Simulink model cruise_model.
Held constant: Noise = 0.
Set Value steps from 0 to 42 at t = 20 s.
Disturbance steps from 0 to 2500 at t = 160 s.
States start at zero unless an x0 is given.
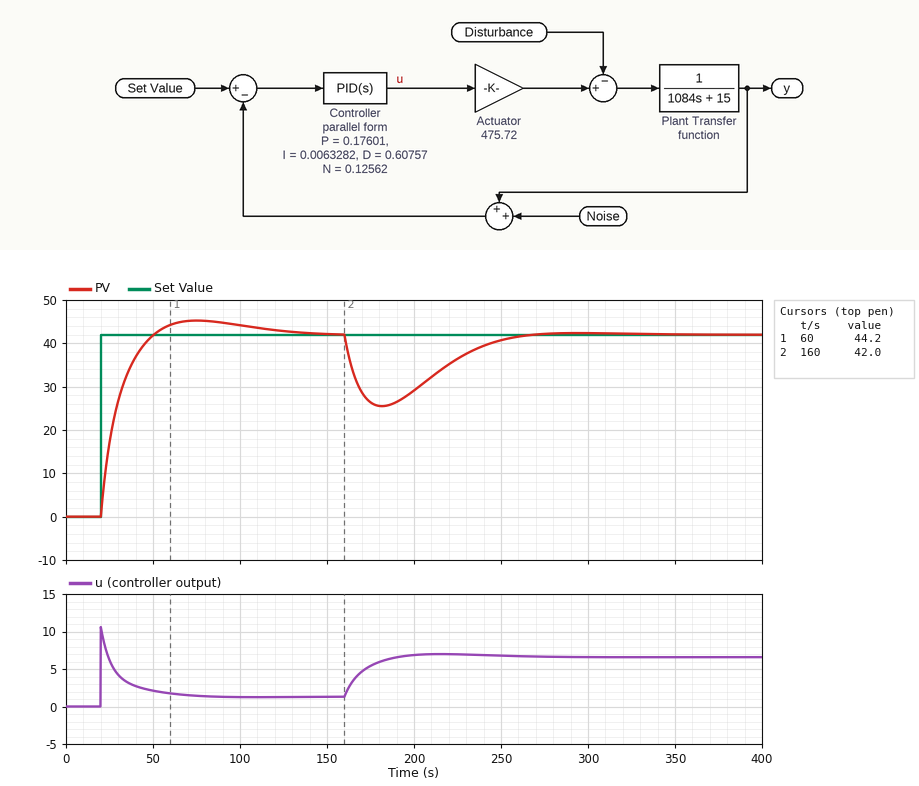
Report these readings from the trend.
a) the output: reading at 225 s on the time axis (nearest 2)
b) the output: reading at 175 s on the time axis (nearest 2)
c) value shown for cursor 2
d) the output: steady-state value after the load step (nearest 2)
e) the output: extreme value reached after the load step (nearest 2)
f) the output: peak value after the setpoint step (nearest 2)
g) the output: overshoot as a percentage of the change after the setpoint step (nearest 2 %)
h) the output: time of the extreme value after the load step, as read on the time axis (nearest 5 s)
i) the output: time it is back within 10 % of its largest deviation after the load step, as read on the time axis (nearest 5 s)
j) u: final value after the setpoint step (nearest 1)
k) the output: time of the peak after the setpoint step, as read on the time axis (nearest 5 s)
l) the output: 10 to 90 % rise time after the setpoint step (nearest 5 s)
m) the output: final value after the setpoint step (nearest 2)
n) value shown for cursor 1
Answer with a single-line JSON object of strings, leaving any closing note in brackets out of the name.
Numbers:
{"the output: reading at 225 s on the time axis": "36", "the output: reading at 175 s on the time axis": "26", "value shown for cursor 2": "42.0", "the output: steady-state value after the load step": "42", "the output: extreme value reached after the load step": "26", "the output: peak value after the setpoint step": "46", "the output: overshoot as a percentage of the change after the setpoint step": "8 %", "the output: time of the extreme value after the load step, as read on the time axis": "180 s", "the output: time it is back within 10 % of its largest deviation after the load step, as read on the time axis": "245 s", "u: final value after the setpoint step": "1", "the output: time of the peak after the setpoint step, as read on the time axis": "75 s", "the output: 10 to 90 % rise time after the setpoint step": "20 s", "the output: final value after the setpoint step": "42", "value shown for cursor 1": "44.2"}
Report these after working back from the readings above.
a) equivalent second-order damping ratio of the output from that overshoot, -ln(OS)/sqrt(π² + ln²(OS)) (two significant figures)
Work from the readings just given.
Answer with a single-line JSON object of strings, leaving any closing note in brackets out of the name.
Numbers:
{"equivalent second-order damping ratio of the output from that overshoot, -ln(OS)/sqrt(π² + ln²(OS))": "0.63"}
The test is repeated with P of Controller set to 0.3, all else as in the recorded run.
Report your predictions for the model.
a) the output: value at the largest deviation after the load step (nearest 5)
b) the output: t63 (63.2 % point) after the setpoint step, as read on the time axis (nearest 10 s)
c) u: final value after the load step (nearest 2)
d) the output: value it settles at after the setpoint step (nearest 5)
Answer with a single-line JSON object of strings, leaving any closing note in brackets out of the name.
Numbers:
{"the output: value at the largest deviation after the load step": "30", "the output: t63 (63.2 % point) after the setpoint step, as read on the time axis": "30 s", "u: final value after the load step": "6", "the output: value it settles at after the setpoint step": "40"}
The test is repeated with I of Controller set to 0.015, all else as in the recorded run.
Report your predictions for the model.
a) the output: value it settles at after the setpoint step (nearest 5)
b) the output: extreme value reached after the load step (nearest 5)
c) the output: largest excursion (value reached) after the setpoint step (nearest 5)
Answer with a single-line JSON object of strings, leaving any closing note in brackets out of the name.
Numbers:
{"the output: value it settles at after the setpoint step": "40", "the output: extreme value reached after the load step": "30", "the output: largest excursion (value reached) after the setpoint step": "50"}
